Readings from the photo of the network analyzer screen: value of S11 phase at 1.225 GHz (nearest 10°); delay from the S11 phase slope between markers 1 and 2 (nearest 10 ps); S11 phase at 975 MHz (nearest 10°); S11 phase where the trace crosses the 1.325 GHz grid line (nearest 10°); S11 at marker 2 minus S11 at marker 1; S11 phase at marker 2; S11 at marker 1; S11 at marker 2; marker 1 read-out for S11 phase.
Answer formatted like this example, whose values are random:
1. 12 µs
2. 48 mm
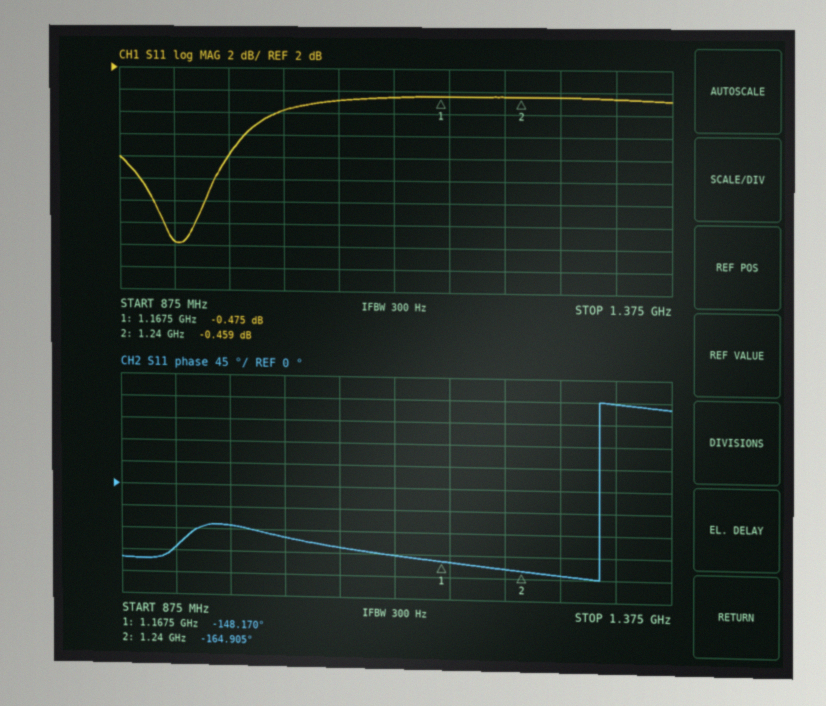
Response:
1. -160°
2. 640 ps
3. -80°
4. 180°
5. 0.016 dB
6. -164.905°
7. -0.475 dB
8. -0.459 dB
9. -148.170°
